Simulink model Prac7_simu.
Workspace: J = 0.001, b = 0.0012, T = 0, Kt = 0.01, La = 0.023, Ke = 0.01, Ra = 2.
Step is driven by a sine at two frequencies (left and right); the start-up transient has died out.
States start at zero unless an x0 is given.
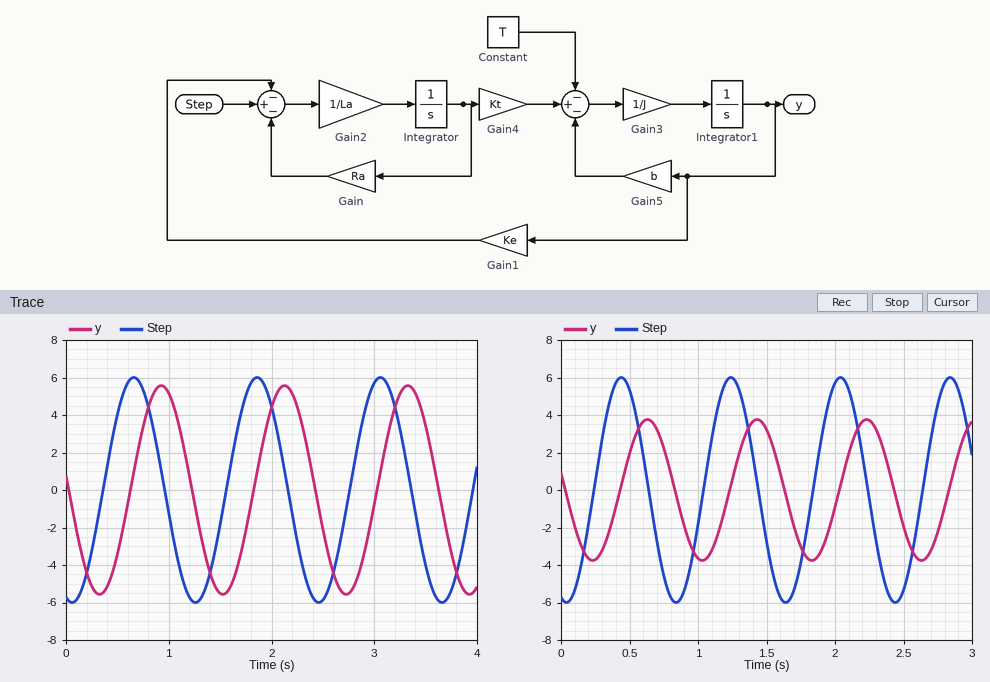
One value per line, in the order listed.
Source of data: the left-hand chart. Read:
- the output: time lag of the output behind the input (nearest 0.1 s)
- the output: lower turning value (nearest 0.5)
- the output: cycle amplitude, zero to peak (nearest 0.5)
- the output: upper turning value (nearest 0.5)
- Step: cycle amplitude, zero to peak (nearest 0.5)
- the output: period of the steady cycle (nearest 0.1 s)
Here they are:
0.3 s
-5.5
5.5
5.5
6.0
1.2 s
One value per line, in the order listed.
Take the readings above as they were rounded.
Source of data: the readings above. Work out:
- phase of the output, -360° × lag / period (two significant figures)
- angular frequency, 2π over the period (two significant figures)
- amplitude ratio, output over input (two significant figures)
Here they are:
-90°
5.2 rad/s
0.92
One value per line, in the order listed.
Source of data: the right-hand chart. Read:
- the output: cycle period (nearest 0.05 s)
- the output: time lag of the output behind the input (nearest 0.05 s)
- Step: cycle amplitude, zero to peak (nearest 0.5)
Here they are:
0.80 s
0.20 s
6.0
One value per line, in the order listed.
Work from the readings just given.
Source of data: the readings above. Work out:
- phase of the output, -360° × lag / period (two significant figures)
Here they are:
-90°
